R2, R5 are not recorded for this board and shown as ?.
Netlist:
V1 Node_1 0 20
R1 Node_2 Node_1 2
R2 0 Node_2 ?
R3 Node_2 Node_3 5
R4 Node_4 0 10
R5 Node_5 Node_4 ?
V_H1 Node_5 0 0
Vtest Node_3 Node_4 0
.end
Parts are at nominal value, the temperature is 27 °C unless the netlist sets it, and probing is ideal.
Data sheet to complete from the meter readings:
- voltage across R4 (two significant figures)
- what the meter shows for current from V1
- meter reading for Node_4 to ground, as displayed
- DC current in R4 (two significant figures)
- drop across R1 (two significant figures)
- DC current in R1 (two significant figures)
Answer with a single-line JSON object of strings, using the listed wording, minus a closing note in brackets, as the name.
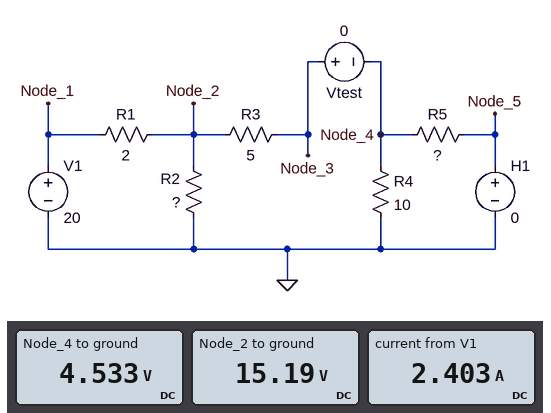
{"voltage across R4": "4.5 V", "what the meter shows for current from V1": "2.403 A", "meter reading for Node_4 to ground, as displayed": "4.533 V", "DC current in R4": "450 mA", "drop across R1": "4.8 V", "DC current in R1": "2.4 A"}
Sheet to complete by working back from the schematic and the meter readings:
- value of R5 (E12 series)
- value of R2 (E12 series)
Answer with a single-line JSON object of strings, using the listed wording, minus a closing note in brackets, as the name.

{"value of R5": "2.7 Ω", "value of R2": "56 Ω"}
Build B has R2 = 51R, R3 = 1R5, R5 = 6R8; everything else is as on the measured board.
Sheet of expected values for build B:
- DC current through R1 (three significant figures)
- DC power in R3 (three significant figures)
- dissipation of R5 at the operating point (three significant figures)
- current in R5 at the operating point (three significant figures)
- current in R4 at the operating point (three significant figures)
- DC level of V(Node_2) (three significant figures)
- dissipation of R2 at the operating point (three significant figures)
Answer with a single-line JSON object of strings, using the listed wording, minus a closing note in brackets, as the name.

{"DC current through R1": "2.86 A", "DC power in R3": "9.95 W", "dissipation of R5 at the operating point": "16.0 W", "current in R5 at the operating point": "1.53 A", "current in R4 at the operating point": "1.04 A", "DC level of V(Node_2)": "14.3 V", "dissipation of R2 at the operating point": "4.00 W"}
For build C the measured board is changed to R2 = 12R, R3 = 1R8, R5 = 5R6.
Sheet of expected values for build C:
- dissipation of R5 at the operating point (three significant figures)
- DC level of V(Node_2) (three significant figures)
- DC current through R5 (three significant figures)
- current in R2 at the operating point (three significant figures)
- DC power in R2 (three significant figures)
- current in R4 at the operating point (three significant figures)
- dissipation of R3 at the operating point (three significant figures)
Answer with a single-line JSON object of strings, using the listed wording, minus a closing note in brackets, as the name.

{"dissipation of R5 at the operating point": "13.4 W", "DC level of V(Node_2)": "13.0 V", "DC current through R5": "1.55 A", "current in R2 at the operating point": "1.08 A", "DC power in R2": "14.1 W", "current in R4 at the operating point": "866 mA", "dissipation of R3 at the operating point": "10.5 W"}
